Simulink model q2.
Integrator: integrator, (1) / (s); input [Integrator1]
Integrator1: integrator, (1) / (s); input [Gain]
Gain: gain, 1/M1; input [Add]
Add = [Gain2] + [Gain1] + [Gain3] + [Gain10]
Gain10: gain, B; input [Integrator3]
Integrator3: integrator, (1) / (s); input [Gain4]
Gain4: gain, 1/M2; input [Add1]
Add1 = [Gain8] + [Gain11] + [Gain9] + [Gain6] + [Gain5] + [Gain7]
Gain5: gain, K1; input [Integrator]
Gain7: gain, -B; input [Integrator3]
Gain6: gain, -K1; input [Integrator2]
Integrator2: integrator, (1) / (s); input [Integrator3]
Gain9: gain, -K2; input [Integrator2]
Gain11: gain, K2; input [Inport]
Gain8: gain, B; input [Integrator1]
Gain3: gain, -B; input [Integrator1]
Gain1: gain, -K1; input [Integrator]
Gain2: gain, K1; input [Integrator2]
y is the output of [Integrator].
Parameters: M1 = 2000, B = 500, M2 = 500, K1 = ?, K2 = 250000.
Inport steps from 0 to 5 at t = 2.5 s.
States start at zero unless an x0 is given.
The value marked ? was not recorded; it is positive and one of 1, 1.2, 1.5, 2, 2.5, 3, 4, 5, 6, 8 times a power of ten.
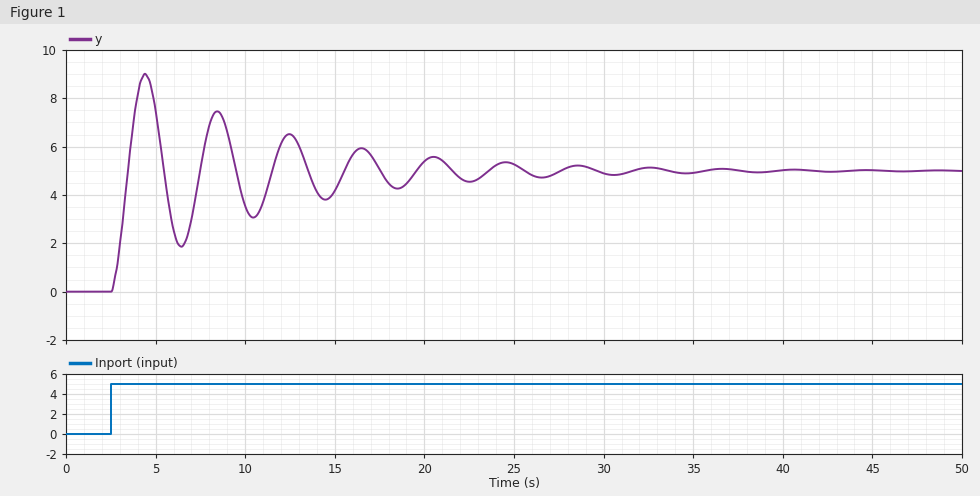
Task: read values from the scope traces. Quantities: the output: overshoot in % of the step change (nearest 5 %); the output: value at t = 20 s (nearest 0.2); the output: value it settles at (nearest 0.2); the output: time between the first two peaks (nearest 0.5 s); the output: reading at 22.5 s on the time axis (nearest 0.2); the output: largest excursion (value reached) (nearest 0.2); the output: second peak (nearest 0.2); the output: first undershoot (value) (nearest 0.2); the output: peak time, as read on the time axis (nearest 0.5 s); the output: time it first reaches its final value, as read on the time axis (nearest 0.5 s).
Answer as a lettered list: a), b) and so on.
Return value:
a) 80 %
b) 5.4
c) 5.0
d) 4.0 s
e) 4.6
f) 9.0
g) 7.4
h) 1.8
i) 4.5 s
j) 3.5 s
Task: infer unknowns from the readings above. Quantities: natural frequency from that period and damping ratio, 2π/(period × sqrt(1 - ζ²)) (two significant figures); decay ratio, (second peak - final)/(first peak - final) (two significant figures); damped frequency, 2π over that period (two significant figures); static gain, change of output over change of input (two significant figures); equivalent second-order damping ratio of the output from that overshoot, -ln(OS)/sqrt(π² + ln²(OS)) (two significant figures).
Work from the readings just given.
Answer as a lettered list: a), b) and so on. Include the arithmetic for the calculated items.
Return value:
a) 2π / (4 × sqrt(1 - 0.071²)) = 1.6 rad/s
b) (7.4 - 5) / (9 - 5) = 0.60
c) 2π / 4 = 1.6 rad/s
d) (5 - 0) / (5 - 0) = 1.0
e) ln(0.8) = -0.223; 0.223 / sqrt(9.870 + 0.050) = 0.071
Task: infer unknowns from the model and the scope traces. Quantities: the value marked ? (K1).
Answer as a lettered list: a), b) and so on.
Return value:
a) 5000
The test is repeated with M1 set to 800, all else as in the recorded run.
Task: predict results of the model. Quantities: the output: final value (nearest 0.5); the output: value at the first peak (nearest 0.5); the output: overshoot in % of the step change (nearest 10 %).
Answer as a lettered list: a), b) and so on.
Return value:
a) 5.0
b) 8.5
c) 70 %
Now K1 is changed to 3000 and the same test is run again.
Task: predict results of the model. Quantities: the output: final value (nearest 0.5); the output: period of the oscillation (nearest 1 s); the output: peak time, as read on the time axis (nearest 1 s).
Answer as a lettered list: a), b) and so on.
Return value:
a) 5.0
b) 5 s
c) 5 s
